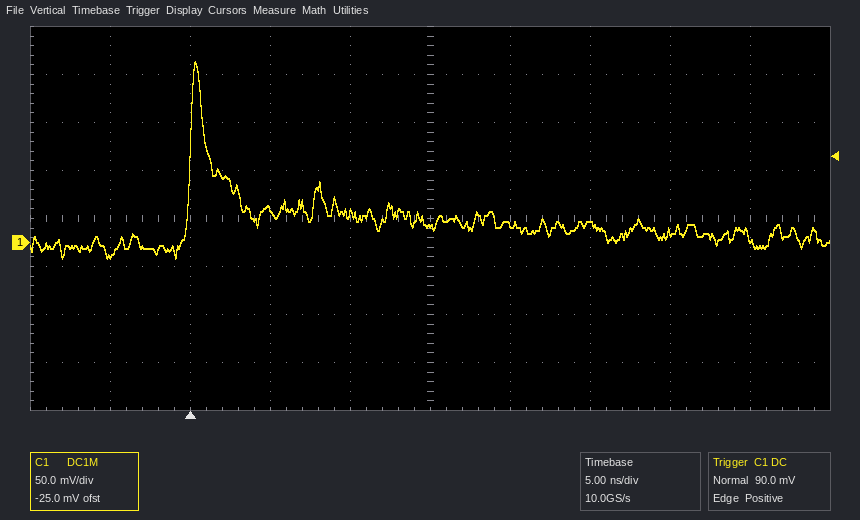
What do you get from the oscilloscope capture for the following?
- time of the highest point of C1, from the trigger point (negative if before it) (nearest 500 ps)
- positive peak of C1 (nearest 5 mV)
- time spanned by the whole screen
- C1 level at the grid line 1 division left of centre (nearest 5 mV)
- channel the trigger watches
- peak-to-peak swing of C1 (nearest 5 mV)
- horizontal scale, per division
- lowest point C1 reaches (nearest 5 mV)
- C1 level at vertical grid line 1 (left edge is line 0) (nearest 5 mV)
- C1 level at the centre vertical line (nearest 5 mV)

+500 ps
190 mV
50 ns
30 mV
C1
205 mV
5 ns
-15 mV
-15 mV
15 mV
